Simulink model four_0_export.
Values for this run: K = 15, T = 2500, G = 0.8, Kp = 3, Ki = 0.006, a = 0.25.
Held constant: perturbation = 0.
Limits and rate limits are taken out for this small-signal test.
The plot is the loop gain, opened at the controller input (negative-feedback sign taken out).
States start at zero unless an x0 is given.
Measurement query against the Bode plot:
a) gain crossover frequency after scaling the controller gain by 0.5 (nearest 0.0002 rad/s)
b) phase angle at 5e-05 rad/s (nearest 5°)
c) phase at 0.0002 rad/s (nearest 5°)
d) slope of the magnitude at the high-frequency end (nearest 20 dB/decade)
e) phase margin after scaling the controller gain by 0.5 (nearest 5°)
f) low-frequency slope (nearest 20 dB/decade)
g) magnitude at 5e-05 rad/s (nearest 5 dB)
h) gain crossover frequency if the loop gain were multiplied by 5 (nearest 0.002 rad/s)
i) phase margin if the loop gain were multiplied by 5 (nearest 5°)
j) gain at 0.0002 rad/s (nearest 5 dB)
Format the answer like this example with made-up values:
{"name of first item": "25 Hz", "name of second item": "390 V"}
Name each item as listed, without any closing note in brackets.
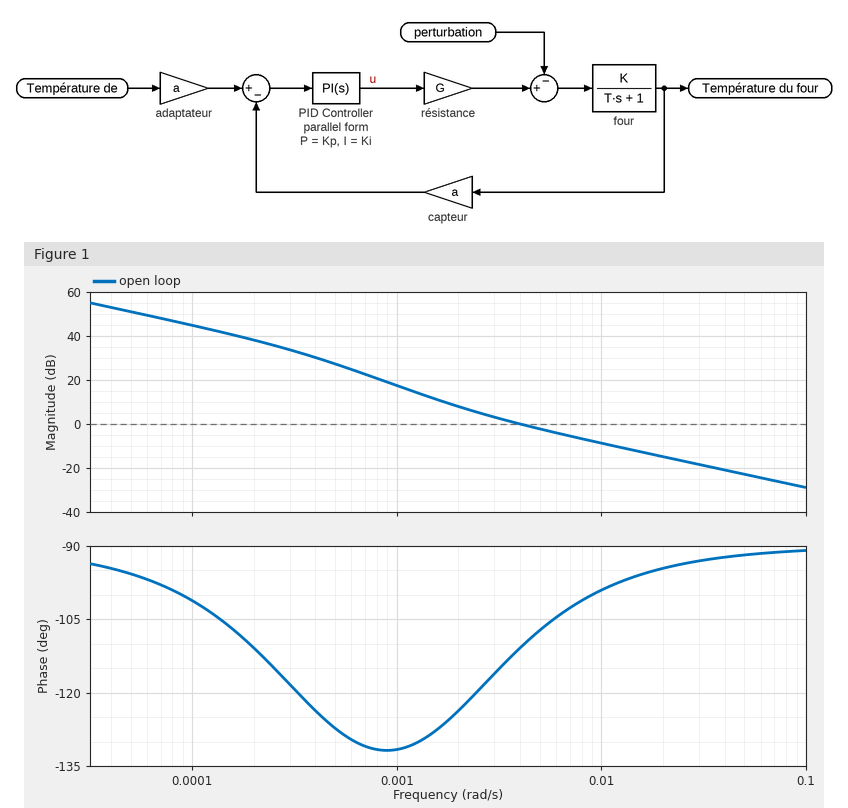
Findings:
{"gain crossover frequency after scaling the controller gain by 0.5": "0.0024 rad/s", "phase angle at 5e-05 rad/s": "-95°", "phase at 0.0002 rad/s": "-110°", "slope of the magnitude at the high-frequency end": "-20 dB/decade", "phase margin after scaling the controller gain by 0.5": "60°", "low-frequency slope": "-20 dB/decade", "magnitude at 5e-05 rad/s": "50 dB", "gain crossover frequency if the loop gain were multiplied by 5": "0.018 rad/s", "phase margin if the loop gain were multiplied by 5": "85°", "gain at 0.0002 rad/s": "40 dB"}
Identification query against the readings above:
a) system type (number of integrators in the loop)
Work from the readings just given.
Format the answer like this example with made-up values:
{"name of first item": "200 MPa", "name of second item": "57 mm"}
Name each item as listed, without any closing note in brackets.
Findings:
{"system type": "1"}
